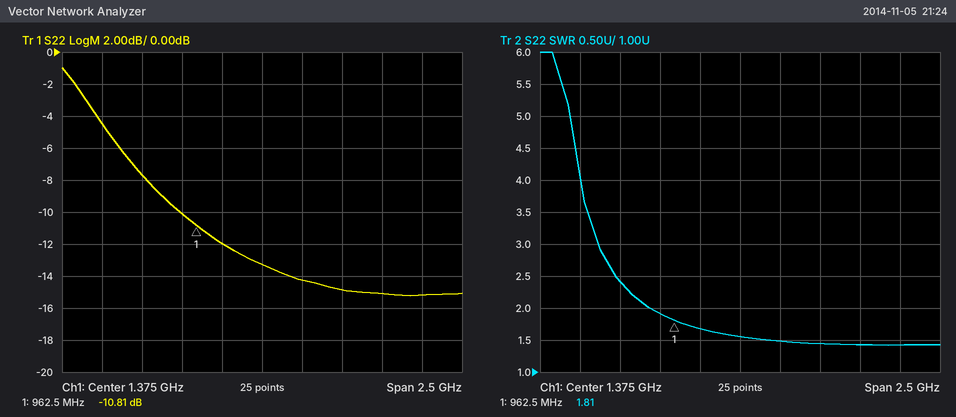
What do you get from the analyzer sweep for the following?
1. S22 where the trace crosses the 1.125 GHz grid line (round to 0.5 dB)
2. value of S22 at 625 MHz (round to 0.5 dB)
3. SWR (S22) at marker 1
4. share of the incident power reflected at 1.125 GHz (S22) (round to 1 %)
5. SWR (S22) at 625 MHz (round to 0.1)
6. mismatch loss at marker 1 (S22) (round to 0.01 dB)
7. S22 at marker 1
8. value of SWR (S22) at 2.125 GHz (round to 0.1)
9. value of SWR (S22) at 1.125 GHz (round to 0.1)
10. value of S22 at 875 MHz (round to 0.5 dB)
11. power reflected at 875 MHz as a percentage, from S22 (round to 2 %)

-12.0 dB
-7.5 dB
1.81
6 %
2.4
0.38 dB
-10.81 dB
1.4
1.7
-10.0 dB
10 %
